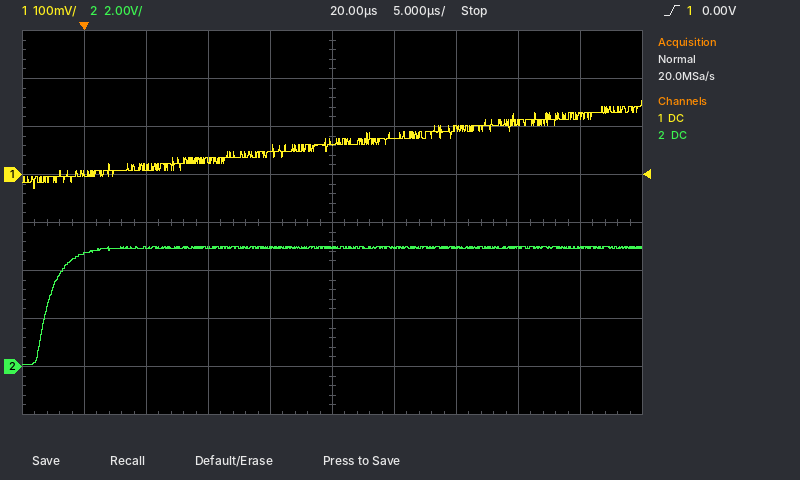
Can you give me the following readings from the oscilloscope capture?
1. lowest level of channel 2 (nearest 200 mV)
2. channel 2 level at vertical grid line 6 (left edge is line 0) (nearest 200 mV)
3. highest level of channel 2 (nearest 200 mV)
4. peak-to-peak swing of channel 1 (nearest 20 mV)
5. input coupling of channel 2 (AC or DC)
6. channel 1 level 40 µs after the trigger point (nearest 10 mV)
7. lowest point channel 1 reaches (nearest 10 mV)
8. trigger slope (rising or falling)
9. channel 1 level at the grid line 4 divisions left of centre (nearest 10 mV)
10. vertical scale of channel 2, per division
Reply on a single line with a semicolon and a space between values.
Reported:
0.0 V; 5.0 V; 5.0 V; 180 mV; DC; 120 mV; -30 mV; rising; 0 mV; 2 V
